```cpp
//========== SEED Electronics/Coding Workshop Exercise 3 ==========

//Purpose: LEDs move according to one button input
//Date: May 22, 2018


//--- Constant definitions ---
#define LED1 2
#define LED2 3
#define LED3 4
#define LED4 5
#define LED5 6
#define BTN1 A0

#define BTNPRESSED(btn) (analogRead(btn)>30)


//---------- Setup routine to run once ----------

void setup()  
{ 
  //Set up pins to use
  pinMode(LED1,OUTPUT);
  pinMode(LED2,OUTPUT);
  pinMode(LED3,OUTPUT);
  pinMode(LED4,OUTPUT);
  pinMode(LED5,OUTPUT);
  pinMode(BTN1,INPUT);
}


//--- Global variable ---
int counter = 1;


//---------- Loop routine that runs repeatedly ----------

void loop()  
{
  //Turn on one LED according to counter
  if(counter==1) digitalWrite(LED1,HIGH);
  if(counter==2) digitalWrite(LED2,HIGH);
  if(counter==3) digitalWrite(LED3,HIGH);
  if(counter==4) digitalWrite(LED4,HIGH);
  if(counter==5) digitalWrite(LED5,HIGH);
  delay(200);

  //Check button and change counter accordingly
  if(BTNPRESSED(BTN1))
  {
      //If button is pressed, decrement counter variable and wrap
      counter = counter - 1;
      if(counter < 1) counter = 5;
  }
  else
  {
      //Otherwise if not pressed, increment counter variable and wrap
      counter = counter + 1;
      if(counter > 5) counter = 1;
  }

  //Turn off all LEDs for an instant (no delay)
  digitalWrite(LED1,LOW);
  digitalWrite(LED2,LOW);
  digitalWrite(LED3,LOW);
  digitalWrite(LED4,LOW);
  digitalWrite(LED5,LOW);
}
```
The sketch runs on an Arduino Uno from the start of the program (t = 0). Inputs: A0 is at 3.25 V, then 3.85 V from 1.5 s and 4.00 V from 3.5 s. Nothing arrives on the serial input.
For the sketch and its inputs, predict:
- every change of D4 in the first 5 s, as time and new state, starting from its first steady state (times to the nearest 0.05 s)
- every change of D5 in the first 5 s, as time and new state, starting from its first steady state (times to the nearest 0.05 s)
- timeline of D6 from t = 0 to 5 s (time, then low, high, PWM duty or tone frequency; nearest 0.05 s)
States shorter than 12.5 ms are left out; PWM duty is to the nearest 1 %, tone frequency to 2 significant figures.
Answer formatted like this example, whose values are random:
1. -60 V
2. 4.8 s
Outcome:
1. 0 s low; 0.6 s high; 0.8 s low; 1.6 s high; 1.8 s low; 2.6 s high; 2.8 s low; 3.6 s high; 3.8 s low; 4.6 s high; 4.8 s low
2. 0 s low; 0.4 s high; 0.6 s low; 1.4 s high; 1.6 s low; 2.4 s high; 2.6 s low; 3.4 s high; 3.6 s low; 4.4 s high; 4.6 s low
3. 0 s low; 0.2 s high; 0.4 s low; 1.2 s high; 1.4 s low; 2.2 s high; 2.4 s low; 3.2 s high; 3.4 s low; 4.2 s high; 4.4 s low
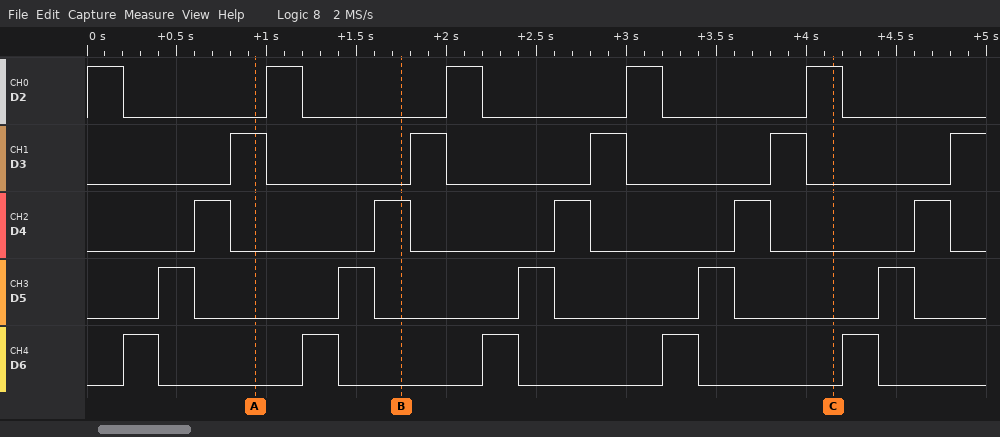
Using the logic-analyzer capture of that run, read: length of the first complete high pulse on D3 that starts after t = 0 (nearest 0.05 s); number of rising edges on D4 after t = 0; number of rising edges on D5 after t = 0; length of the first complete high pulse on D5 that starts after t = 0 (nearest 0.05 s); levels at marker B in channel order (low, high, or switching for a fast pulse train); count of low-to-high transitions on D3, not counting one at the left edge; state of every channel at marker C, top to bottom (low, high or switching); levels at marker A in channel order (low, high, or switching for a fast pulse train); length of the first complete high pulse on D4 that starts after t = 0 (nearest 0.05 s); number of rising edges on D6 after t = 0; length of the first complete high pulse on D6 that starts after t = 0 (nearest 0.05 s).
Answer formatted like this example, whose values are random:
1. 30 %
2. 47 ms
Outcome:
1. 0.20 s
2. 5
3. 5
4. 0.20 s
5. D2 low, D3 low, D4 high, D5 low, D6 low
6. 5
7. D2 high, D3 low, D4 low, D5 low, D6 low
8. D2 low, D3 high, D4 low, D5 low, D6 low
9. 0.20 s
10. 5
11. 0.20 s
